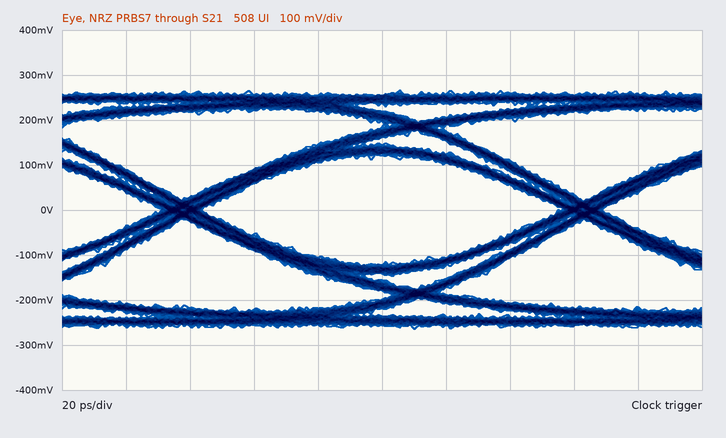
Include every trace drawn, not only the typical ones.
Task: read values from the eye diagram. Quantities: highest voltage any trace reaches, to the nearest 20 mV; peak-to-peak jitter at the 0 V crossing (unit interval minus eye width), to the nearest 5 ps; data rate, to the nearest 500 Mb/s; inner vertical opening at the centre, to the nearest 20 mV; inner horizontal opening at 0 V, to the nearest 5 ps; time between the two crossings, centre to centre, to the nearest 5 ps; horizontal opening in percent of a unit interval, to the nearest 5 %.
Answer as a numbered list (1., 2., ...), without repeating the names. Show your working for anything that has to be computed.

1. 260 mV
2. 15 ps
3. 8.0 Gb/s
4. 240 mV
5. 110 ps
6. 125 ps
7. 110 ps / 125 ps ≈ 88.0 %, so 90 % to the nearest 5 %
